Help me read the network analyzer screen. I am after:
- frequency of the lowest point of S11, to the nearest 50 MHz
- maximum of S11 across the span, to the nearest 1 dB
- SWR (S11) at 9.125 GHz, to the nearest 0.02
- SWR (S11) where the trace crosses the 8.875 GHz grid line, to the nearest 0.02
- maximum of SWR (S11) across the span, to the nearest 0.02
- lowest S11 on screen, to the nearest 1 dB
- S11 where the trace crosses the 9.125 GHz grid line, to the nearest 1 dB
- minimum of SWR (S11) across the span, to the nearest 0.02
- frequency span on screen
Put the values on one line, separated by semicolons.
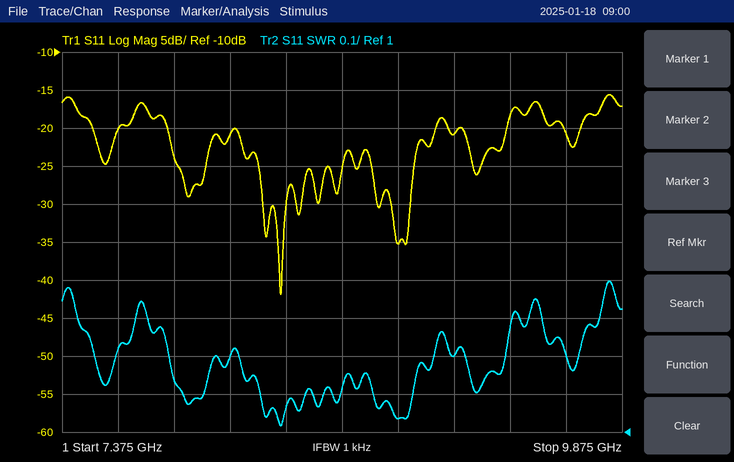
8.35 GHz; -16 dB; 1.20; 1.04; 1.40; -42 dB; -21 dB; 1.02; 2.5 GHz
